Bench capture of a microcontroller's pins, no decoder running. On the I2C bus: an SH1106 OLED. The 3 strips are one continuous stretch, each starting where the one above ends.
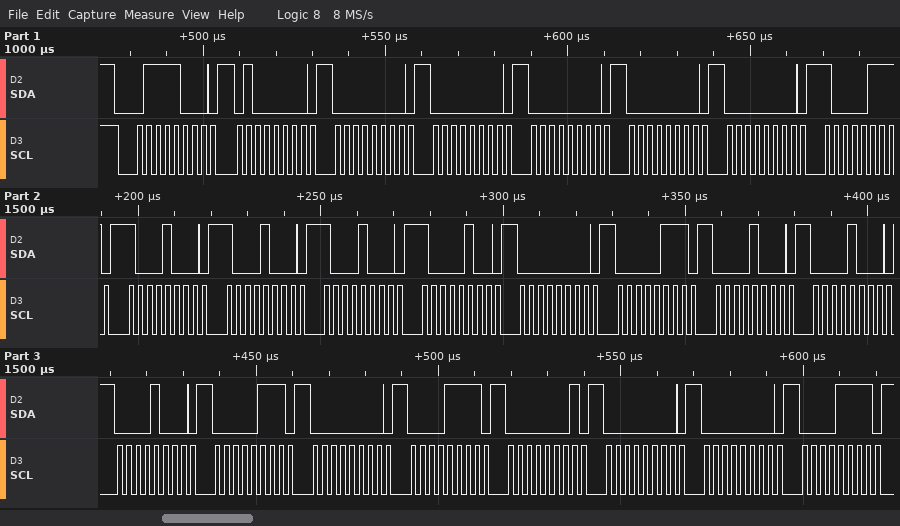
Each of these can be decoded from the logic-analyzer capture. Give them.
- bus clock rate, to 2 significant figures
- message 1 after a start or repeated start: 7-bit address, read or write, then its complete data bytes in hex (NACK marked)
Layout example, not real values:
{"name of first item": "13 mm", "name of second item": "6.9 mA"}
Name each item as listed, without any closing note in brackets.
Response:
{"bus clock rate, to 2 significant figures": "400 kHz", "message 1 after a start or repeated start: 7-bit address, read or write, then its complete data bytes in hex": "0x3C write: 40 00 00 00 00 00 87 88 88 88 84 00 07 08 08 08 07 00 0F 01 00 00 0F"}
